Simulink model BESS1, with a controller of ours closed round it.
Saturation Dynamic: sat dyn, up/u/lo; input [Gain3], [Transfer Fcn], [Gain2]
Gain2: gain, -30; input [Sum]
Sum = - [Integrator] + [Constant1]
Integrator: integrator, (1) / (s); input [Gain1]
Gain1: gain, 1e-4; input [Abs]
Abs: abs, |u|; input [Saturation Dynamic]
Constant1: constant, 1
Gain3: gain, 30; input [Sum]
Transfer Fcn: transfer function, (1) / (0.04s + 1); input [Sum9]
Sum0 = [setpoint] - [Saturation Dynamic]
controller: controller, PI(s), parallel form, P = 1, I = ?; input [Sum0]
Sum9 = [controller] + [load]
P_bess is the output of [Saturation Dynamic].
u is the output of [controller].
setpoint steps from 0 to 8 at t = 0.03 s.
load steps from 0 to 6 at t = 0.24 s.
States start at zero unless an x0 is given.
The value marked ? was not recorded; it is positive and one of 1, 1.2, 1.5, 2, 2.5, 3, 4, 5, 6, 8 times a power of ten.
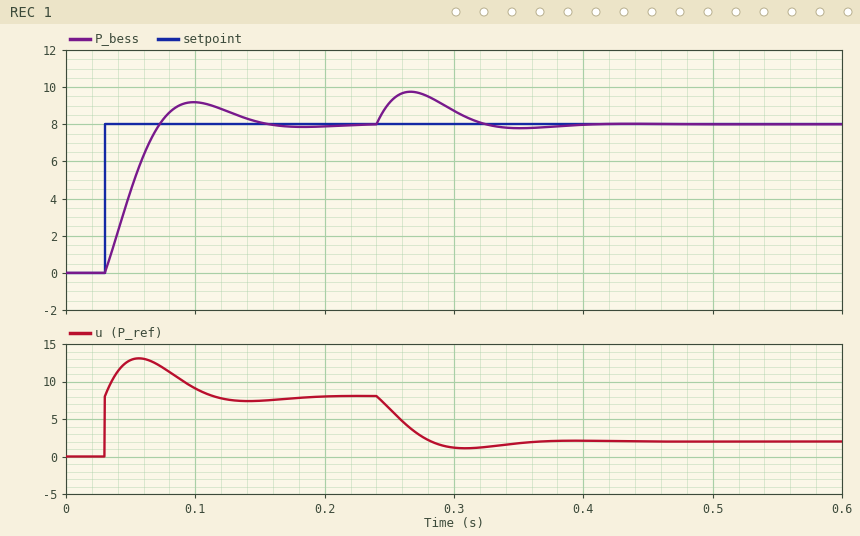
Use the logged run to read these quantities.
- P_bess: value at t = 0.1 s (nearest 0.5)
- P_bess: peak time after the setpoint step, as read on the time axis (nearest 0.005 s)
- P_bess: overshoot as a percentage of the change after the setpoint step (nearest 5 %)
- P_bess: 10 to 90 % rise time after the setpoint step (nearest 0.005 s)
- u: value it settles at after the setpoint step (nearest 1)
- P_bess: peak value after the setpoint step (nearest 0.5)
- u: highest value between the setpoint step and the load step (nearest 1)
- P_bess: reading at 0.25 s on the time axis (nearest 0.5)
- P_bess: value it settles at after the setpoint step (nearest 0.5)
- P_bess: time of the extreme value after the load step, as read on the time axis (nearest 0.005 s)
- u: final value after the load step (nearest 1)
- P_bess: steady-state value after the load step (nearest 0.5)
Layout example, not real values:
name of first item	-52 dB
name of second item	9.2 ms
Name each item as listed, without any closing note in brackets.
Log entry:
P_bess: value at t = 0.1 s	9.0
P_bess: peak time after the setpoint step, as read on the time axis	0.100 s
P_bess: overshoot as a percentage of the change after the setpoint step	15 %
P_bess: 10 to 90 % rise time after the setpoint step	0.030 s
u: value it settles at after the setpoint step	8
P_bess: peak value after the setpoint step	9.0
u: highest value between the setpoint step and the load step	13
P_bess: reading at 0.25 s on the time axis	9.0
P_bess: value it settles at after the setpoint step	8.0
P_bess: time of the extreme value after the load step, as read on the time axis	0.265 s
u: final value after the load step	2
P_bess: steady-state value after the load step	8.0
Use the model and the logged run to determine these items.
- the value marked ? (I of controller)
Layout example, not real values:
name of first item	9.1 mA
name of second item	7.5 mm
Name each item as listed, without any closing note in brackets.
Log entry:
the value marked ?	80
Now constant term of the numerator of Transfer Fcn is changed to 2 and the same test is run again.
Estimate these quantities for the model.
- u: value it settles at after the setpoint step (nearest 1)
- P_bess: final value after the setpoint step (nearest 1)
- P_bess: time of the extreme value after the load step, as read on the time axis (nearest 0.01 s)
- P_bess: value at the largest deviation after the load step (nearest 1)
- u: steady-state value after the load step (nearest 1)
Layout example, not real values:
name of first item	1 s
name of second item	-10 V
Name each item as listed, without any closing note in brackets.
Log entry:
u: value it settles at after the setpoint step	4
P_bess: final value after the setpoint step	8
P_bess: time of the extreme value after the load step, as read on the time axis	0.26 s
P_bess: value at the largest deviation after the load step	10
u: steady-state value after the load step	-2
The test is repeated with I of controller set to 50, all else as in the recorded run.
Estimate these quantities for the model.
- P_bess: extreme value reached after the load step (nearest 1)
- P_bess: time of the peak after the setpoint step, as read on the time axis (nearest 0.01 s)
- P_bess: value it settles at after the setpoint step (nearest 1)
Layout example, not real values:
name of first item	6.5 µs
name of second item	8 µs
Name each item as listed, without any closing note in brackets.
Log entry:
P_bess: extreme value reached after the load step	10
P_bess: time of the peak after the setpoint step, as read on the time axis	0.12 s
P_bess: value it settles at after the setpoint step	8
